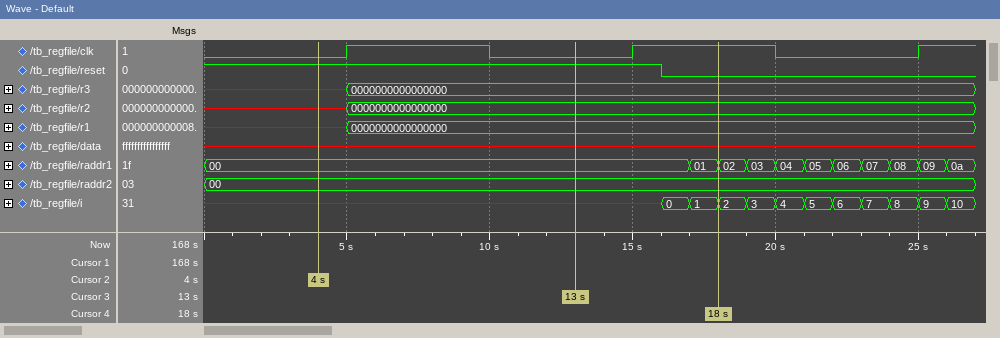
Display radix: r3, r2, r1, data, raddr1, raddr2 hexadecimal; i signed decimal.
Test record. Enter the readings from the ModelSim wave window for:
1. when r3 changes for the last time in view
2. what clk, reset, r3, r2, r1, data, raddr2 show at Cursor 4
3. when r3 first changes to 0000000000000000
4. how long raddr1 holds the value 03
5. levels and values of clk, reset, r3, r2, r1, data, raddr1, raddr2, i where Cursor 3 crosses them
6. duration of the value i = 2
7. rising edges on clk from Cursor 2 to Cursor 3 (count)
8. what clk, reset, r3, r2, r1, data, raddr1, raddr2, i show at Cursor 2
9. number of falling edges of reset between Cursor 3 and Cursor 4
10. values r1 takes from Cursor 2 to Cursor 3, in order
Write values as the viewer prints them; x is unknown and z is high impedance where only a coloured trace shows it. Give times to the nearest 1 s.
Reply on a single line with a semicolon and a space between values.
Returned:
5 s; clk=1, reset=0, r3=0000000000000000, r2=0000000000000000, r1=0000000000000000, data=x, raddr2=00; 5 s; 1 s; clk=0, reset=1, r3=0000000000000000, r2=0000000000000000, r1=0000000000000000, data=x, raddr1=00, raddr2=00, i=x; 1 s; 1; clk=0, reset=1, r3=x, r2=x, r1=x, data=x, raddr1=00, raddr2=00, i=x; 1; x, 0000000000000000
